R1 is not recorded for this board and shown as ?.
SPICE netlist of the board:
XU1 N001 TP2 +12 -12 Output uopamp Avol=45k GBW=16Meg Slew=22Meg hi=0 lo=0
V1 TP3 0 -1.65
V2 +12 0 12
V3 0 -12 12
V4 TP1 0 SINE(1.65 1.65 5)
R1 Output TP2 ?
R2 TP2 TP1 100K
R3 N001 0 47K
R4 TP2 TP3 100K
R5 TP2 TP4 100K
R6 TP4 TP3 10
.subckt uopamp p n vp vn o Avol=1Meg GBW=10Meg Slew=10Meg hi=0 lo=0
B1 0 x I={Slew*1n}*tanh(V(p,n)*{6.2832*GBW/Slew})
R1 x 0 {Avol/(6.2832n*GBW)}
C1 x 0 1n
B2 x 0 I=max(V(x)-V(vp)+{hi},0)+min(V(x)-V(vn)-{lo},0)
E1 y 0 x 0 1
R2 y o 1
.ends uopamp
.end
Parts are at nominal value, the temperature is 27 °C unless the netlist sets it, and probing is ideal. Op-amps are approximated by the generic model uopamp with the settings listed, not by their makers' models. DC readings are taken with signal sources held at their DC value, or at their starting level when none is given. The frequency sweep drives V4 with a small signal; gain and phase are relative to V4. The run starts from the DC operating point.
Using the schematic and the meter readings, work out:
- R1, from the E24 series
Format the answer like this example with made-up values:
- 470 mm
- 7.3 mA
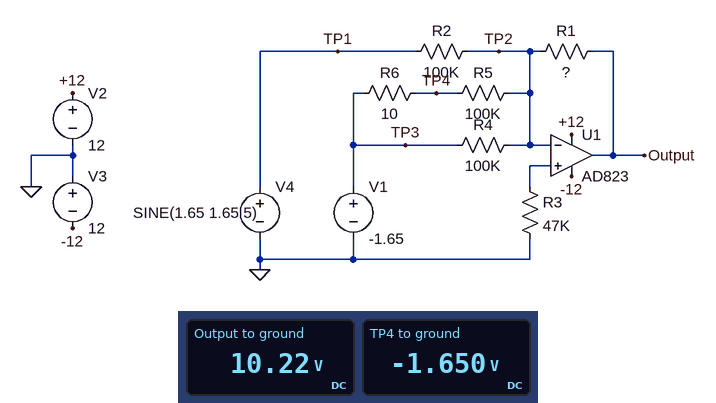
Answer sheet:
- 620 kΩ
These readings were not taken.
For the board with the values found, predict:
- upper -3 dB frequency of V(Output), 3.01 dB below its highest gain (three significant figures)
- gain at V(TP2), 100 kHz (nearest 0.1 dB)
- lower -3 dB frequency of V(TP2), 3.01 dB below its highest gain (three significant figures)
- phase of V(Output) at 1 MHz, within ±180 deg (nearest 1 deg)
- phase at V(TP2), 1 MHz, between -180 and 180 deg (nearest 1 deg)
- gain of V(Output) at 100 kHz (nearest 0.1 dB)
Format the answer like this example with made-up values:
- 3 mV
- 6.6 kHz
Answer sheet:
- 817 kHz
- -28.3 dB
- 817 kHz
- 129 deg
- 39 deg
- 15.8 dB
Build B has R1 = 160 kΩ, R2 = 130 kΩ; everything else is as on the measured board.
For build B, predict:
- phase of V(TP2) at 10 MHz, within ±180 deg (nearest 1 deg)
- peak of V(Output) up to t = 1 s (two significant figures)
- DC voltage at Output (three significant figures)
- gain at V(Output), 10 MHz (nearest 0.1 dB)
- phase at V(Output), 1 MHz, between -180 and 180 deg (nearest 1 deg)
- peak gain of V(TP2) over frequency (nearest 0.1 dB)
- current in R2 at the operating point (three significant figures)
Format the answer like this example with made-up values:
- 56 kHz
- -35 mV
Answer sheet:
- 16 deg
- 5.3 V
- 3.25 V
- -9.2 dB
- 161 deg
- -12.9 dB
- 12.7 µA
